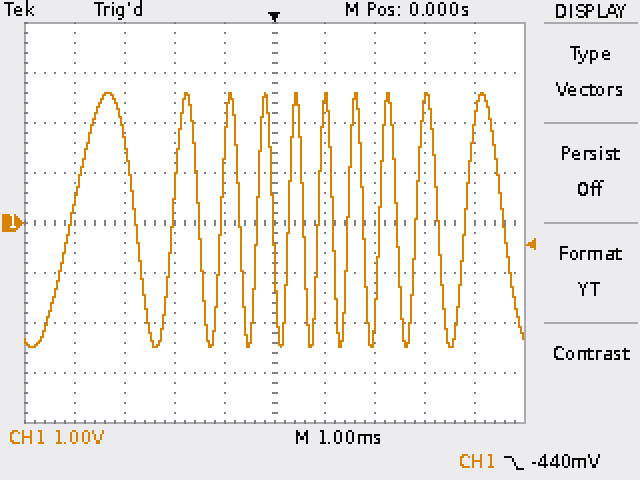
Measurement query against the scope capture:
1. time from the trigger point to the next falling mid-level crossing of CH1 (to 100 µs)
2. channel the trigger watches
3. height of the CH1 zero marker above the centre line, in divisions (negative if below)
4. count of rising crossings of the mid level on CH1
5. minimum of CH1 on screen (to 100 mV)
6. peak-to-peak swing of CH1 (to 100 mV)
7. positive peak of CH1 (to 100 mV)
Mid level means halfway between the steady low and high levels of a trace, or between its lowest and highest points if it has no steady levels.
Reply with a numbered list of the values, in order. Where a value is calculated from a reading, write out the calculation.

1. 600 µs
2. CH1
3. 0.0 div
4. 10
5. -2.5 V
6. 2.6 V − (-2.5 V) = 5.1 V
7. 2.6 V
